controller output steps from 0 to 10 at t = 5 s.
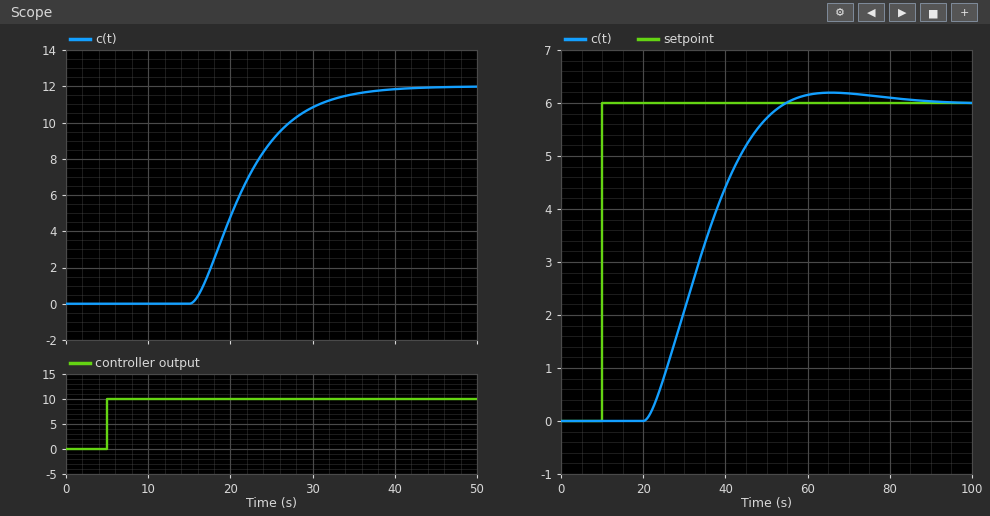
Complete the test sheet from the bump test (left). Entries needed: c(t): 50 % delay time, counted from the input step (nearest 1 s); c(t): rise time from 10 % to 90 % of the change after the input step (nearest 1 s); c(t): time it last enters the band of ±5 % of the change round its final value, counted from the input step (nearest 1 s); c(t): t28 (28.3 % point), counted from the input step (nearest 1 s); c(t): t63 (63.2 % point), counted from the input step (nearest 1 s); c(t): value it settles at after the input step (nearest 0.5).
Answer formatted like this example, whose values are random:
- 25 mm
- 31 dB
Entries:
- 16 s
- 13 s
- 28 s
- 14 s
- 18 s
- 12.0
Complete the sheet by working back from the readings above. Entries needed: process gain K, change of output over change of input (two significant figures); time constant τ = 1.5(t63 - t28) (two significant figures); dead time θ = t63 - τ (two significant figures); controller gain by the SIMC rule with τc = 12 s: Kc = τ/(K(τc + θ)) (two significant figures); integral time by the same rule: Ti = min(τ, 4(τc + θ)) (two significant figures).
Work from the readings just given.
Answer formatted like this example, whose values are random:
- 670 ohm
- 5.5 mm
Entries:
- 1.2
- 6.0 s
- 12 s
- 0.21
- 6.0 s
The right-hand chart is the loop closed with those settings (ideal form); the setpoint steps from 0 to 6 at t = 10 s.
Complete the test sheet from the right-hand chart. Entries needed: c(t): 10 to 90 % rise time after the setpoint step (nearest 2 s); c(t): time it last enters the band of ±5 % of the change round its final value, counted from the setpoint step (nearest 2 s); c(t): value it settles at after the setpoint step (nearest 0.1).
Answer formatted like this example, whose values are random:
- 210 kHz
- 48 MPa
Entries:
- 22 s
- 40 s
- 6.0
